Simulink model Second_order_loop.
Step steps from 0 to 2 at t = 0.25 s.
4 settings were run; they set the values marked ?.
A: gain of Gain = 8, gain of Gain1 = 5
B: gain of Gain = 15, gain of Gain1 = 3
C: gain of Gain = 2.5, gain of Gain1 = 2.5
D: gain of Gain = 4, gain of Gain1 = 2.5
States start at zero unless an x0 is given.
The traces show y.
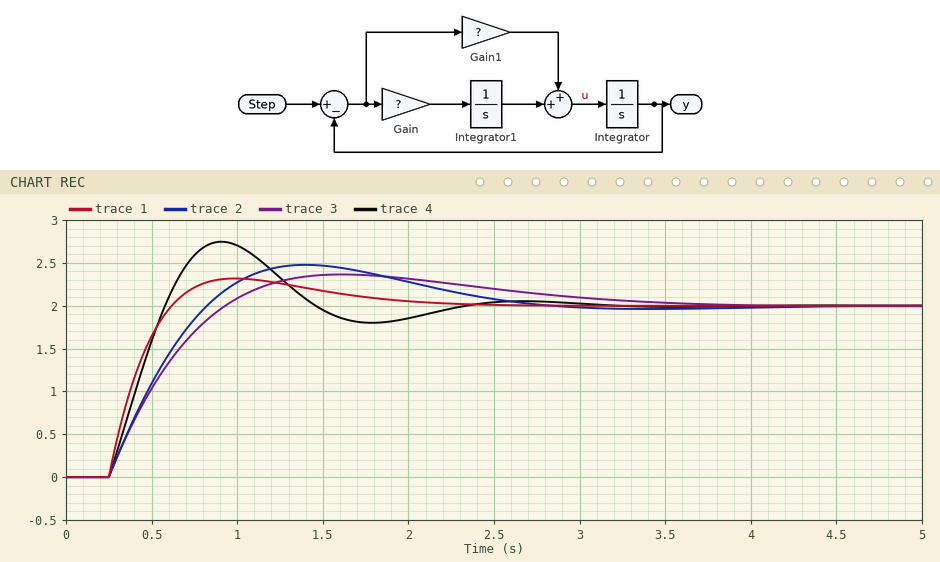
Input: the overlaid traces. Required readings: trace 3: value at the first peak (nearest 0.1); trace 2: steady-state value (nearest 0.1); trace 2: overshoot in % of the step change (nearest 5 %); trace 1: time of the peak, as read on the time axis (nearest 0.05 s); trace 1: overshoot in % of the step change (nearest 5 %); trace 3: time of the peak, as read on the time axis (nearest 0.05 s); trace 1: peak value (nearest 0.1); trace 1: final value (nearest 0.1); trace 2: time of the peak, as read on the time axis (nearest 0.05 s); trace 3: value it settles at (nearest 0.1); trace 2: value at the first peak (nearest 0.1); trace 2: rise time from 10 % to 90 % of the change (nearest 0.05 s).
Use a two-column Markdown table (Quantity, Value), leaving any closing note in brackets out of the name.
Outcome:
| Quantity | Value |
|---|---|
| trace 3: value at the first peak | 2.4 |
| trace 2: steady-state value | 2.0 |
| trace 2: overshoot in % of the step change | 25 % |
| trace 1: time of the peak, as read on the time axis | 1.00 s |
| trace 1: overshoot in % of the step change | 15 % |
| trace 3: time of the peak, as read on the time axis | 1.60 s |
| trace 1: peak value | 2.3 |
| trace 1: final value | 2.0 |
| trace 2: time of the peak, as read on the time axis | 1.40 s |
| trace 3: value it settles at | 2.0 |
| trace 2: value at the first peak | 2.5 |
| trace 2: rise time from 10 % to 90 % of the change | 0.45 s |
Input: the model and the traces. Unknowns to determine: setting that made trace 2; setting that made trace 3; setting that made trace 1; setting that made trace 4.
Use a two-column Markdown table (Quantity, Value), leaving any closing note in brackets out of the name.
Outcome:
| Quantity | Value |
|---|---|
| setting that made trace 2 | D |
| setting that made trace 3 | C |
| setting that made trace 1 | A |
| setting that made trace 4 | B |
